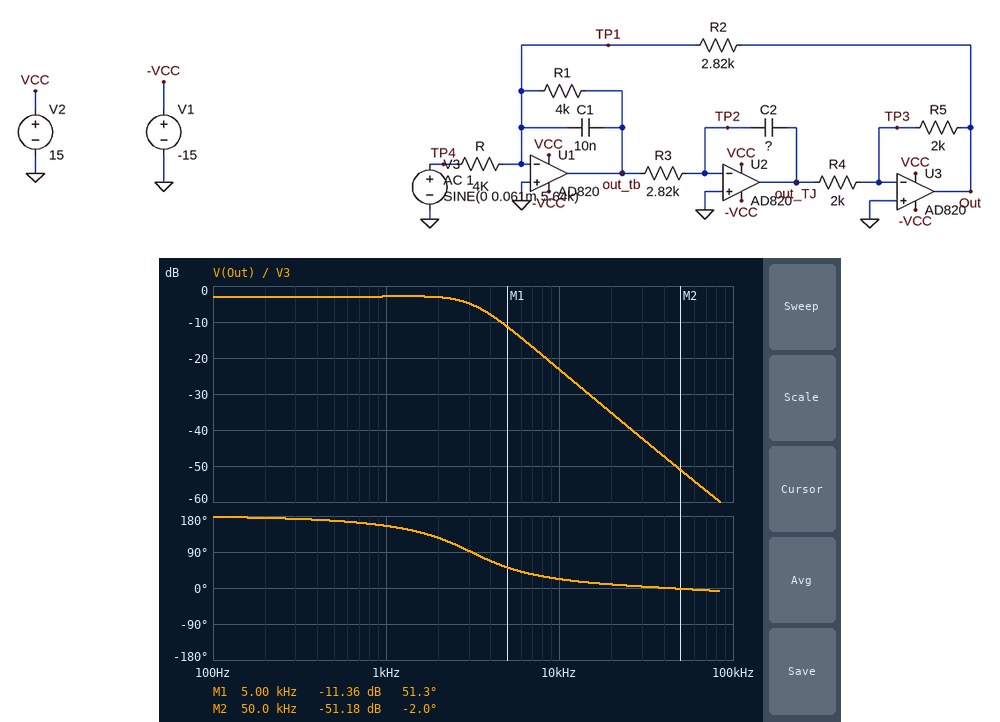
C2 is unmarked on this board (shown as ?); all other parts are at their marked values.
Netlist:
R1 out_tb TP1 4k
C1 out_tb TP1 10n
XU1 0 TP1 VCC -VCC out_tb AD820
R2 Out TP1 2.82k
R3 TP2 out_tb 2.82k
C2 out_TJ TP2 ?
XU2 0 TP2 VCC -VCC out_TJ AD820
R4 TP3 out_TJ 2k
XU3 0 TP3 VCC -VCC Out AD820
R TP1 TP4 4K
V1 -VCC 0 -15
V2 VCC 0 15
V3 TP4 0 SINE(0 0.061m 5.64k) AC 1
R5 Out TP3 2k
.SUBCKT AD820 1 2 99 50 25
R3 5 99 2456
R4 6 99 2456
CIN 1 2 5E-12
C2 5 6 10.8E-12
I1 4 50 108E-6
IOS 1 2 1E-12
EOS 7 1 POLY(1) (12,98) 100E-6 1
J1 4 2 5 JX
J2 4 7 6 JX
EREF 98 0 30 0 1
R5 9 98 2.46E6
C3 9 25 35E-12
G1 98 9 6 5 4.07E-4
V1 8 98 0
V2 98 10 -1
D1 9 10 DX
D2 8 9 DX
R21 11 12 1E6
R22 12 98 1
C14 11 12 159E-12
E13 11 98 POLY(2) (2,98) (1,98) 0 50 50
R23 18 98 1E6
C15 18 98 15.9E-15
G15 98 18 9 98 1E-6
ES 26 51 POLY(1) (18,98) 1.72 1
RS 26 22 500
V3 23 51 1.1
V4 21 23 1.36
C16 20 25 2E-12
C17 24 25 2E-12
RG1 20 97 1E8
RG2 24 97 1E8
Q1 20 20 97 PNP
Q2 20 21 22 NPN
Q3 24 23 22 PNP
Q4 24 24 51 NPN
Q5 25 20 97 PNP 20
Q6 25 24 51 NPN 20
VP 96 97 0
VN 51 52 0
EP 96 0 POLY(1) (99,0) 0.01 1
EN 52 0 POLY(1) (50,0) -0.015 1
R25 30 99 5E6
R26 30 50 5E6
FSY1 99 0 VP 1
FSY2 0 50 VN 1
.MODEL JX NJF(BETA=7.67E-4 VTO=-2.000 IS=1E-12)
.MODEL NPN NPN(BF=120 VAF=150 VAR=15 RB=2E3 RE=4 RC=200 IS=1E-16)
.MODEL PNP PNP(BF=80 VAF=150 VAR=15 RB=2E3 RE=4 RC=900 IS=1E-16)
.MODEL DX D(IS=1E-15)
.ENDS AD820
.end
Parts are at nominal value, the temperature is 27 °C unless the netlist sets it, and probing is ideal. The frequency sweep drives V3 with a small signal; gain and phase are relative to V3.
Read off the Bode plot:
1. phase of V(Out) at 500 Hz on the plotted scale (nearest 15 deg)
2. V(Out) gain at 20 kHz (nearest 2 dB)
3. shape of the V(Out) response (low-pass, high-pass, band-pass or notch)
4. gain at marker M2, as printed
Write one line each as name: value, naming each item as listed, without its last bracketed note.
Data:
phase of V(Out) at 500 Hz on the plotted scale: 165 deg
V(Out) gain at 20 kHz: -36 dB
shape of the V(Out) response: low-pass
gain at marker M2, as printed: -51.18 dB
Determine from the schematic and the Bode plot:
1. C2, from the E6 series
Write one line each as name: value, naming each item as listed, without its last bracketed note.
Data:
C2, from the E6 series: 33 nF
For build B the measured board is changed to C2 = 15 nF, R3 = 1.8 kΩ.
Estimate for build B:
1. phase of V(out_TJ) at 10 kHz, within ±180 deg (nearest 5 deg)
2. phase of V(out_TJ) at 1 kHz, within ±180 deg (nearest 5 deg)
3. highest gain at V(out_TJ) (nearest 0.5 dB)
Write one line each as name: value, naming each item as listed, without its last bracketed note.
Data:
phase of V(out_TJ) at 10 kHz, within ±180 deg: -150 deg
phase of V(out_TJ) at 1 kHz, within ±180 deg: -5 deg
highest gain at V(out_TJ): 1.0 dB
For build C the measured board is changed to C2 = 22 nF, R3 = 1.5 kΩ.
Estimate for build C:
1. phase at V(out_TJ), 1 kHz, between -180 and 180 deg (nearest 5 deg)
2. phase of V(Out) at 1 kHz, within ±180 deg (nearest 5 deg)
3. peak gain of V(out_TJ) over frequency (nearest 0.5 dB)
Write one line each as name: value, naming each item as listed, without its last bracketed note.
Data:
phase at V(out_TJ), 1 kHz, between -180 and 180 deg: -10 deg
phase of V(Out) at 1 kHz, within ±180 deg: 170 deg
peak gain of V(out_TJ) over frequency: 0 dB
